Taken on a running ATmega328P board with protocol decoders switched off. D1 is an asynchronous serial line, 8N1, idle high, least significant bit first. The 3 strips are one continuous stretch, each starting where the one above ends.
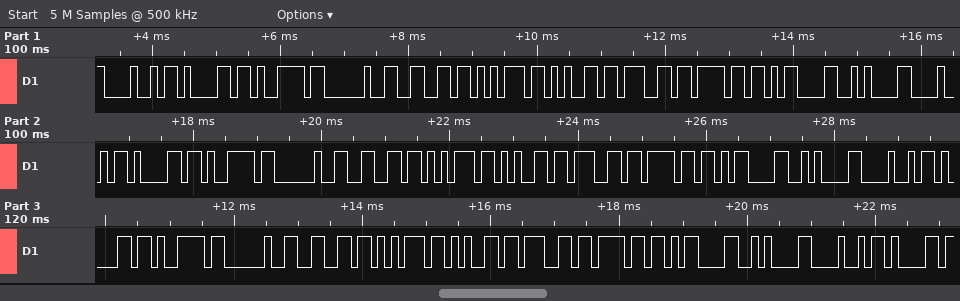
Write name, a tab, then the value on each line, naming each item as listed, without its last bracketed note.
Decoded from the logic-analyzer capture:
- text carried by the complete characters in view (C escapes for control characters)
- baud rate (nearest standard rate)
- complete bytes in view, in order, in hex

text carried by the complete characters in view	"Hay fuego\r\nHay fuego\r\nHay fuego\r\nHa"
baud rate	9600 baud
complete bytes in view, in order, in hex	48 61 79 20 66 75 65 67 6F 0D 0A 48 61 79 20 66 75 65 67 6F 0D 0A 48 61 79 20 66 75 65 67 6F 0D 0A 48 61
